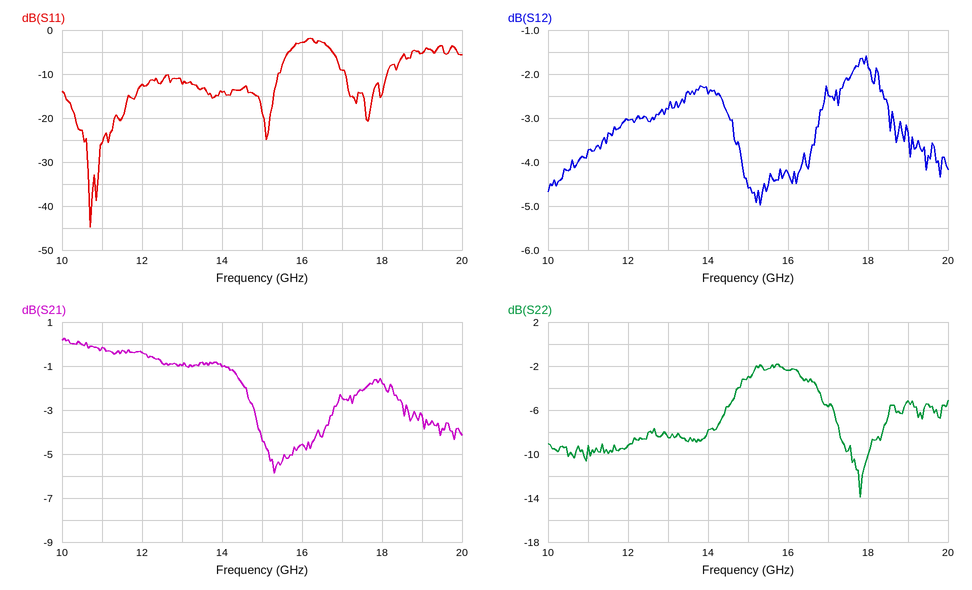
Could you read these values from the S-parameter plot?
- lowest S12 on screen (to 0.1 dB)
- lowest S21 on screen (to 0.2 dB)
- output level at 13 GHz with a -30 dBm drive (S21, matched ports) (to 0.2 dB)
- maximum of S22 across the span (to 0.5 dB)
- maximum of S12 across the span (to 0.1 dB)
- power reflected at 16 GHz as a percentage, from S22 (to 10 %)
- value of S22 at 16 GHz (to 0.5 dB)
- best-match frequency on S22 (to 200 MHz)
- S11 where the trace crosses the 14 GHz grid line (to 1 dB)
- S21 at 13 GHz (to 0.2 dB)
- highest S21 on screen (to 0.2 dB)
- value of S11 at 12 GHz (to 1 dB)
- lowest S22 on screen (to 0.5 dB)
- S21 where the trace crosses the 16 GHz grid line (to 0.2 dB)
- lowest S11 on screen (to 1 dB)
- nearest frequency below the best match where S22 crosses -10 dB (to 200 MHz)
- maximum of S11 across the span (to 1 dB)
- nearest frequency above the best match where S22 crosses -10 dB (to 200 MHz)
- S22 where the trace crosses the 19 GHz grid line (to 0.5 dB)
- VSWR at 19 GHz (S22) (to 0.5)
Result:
-5.0 dB
-5.8 dB
-31.0 dBm
-2.0 dB
-1.6 dB
60 %
-2.5 dB
17.8 GHz
-14 dB
-1.0 dB
0.2 dB
-12 dB
-14.0 dB
-4.6 dB
-45 dB
17.6 GHz
-2 dB
18.0 GHz
-5.0 dB
3.5
